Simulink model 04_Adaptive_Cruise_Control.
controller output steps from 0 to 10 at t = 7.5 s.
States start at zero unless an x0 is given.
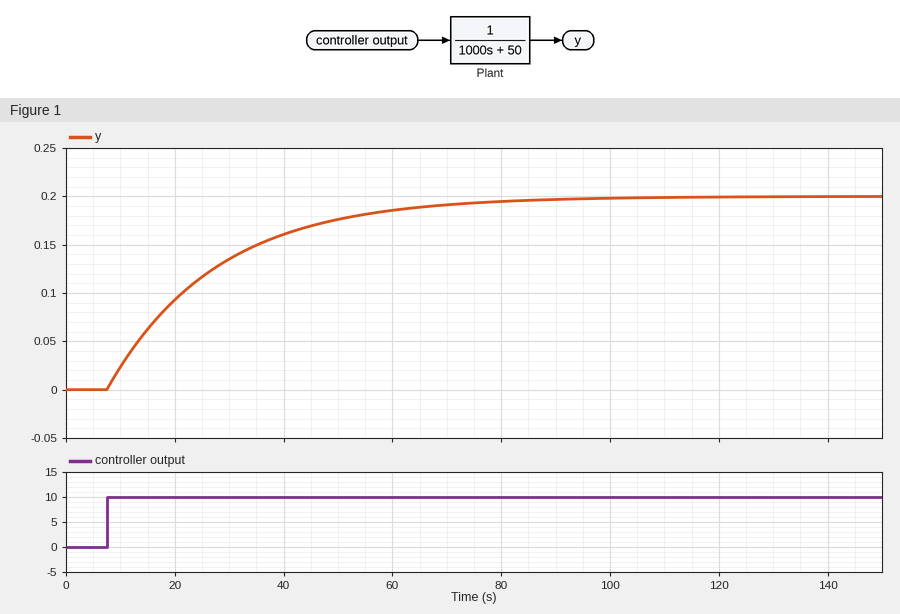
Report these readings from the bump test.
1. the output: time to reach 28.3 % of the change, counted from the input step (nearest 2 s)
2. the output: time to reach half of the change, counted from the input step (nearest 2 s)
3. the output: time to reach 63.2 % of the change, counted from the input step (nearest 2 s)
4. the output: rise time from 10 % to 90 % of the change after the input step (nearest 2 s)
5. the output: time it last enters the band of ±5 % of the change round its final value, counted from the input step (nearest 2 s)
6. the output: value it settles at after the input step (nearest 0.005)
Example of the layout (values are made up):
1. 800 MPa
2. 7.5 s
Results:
1. 6 s
2. 14 s
3. 20 s
4. 44 s
5. 60 s
6. 0.200
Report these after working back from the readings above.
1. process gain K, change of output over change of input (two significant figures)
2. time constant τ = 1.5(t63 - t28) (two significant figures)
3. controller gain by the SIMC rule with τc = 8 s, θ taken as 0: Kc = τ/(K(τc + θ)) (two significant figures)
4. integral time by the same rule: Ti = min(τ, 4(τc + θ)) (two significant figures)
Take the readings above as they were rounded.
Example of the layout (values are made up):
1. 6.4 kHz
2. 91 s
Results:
1. 0.020
2. 21 s
3. 130
4. 21 s
